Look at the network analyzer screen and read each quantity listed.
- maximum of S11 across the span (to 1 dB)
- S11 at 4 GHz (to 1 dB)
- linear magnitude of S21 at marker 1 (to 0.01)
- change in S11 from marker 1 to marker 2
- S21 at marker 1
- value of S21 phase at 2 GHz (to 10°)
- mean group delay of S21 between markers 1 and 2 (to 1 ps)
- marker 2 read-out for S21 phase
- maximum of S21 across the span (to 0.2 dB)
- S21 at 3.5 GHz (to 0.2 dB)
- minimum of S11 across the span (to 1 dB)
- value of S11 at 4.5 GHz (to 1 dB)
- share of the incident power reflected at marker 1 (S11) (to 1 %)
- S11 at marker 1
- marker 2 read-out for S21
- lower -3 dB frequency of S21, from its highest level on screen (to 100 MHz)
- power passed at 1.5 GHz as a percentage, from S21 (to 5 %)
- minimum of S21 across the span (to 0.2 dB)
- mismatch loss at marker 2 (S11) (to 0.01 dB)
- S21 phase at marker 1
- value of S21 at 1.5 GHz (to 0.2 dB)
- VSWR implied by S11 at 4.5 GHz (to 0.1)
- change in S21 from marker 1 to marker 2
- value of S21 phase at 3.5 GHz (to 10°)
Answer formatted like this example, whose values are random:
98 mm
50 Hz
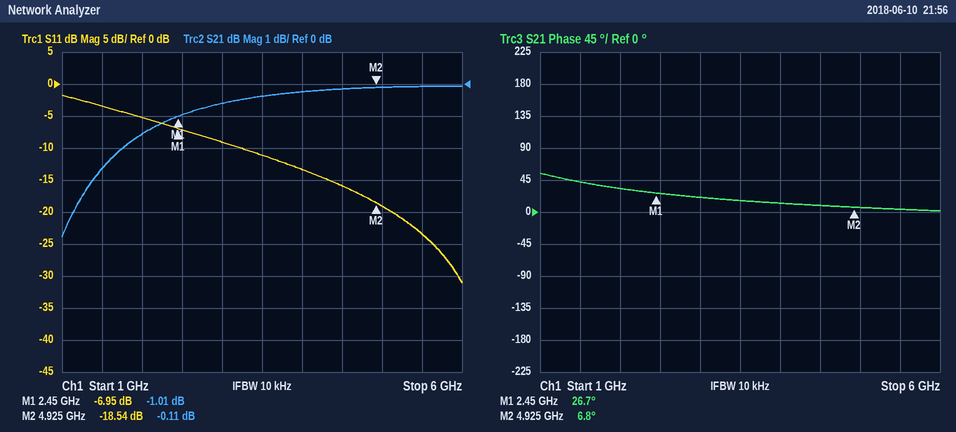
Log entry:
-2 dB
-13 dB
0.89
-11.59 dB
-1.01 dB
30°
22 ps
6.8°
0.0 dB
-0.4 dB
-31 dB
-16 dB
20 %
-6.95 dB
-0.11 dB
1.4 GHz
55 %
-4.8 dB
0.06 dB
26.7°
-2.6 dB
1.4
0.90 dB
20°
